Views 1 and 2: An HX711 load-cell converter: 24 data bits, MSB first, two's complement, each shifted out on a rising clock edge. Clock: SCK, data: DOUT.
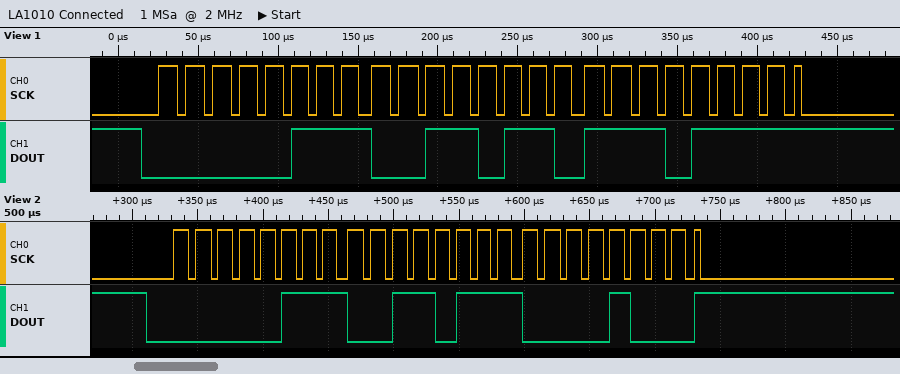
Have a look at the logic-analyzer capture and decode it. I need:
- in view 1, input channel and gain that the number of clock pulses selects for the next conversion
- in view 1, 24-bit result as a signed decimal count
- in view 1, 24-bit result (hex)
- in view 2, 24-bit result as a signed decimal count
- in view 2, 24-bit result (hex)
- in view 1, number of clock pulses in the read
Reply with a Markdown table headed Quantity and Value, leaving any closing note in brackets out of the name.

| Quantity | Value |
|---|---|
| in view 1, input channel and gain that the number of clock pulses selects for the next conversion | channel A, gain 128 |
| in view 1, 24-bit result as a signed decimal count | 472815 |
| in view 1, 24-bit result | 0x0736EF |
| in view 2, 24-bit result as a signed decimal count | 472840 |
| in view 2, 24-bit result | 0x073708 |
| in view 1, number of clock pulses in the read | 25 |
